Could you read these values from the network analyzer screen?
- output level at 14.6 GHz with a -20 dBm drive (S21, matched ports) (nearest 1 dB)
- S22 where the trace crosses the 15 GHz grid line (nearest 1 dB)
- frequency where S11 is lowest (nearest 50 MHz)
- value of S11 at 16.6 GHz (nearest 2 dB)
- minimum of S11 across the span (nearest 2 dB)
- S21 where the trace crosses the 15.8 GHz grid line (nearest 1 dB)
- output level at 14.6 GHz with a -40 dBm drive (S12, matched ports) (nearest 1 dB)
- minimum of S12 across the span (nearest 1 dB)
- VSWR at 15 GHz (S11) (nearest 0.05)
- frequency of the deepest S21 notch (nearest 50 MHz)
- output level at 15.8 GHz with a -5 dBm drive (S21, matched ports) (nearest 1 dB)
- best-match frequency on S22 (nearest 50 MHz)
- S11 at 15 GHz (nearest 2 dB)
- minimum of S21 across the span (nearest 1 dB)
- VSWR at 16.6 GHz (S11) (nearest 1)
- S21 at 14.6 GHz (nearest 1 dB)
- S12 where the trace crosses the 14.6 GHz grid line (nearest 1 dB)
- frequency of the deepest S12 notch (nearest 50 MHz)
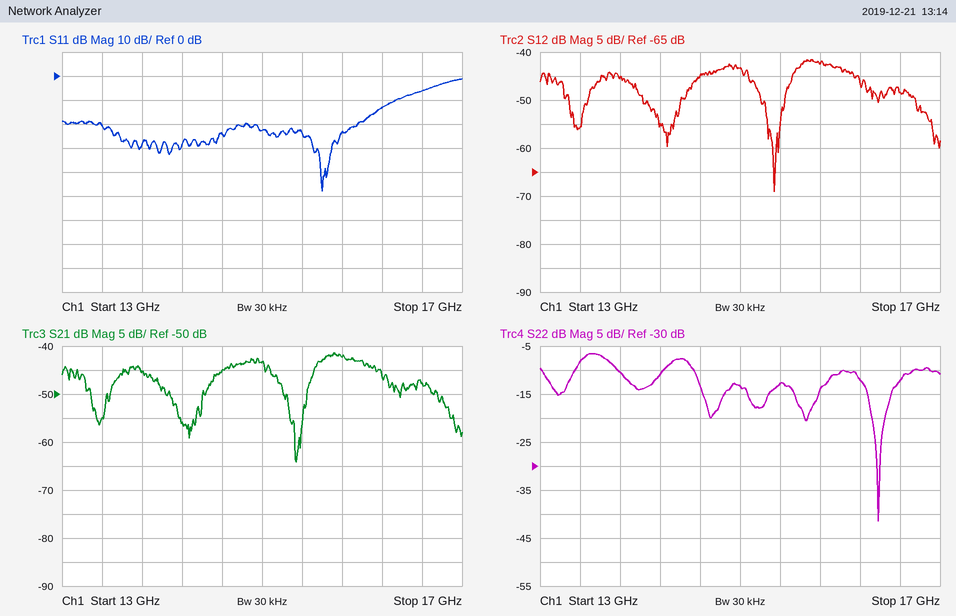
-65 dBm
-13 dB
15.60 GHz
-6 dB
-48 dB
-42 dB
-85 dBm
-69 dB
1.15
15.35 GHz
-47 dBm
16.40 GHz
-22 dB
-64 dB
3
-45 dB
-45 dB
15.35 GHz
